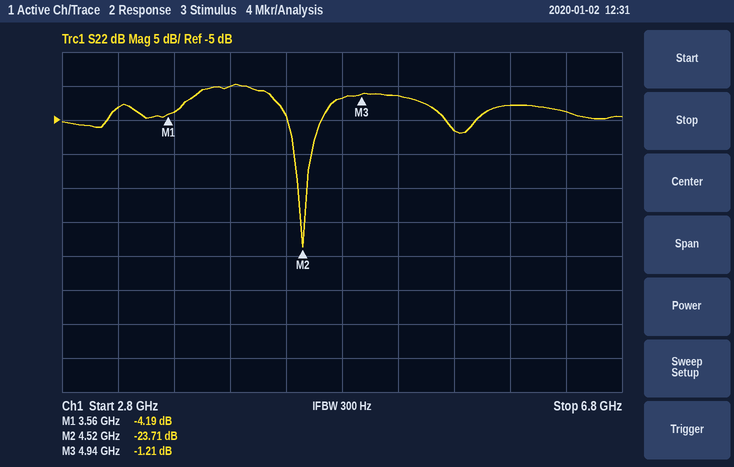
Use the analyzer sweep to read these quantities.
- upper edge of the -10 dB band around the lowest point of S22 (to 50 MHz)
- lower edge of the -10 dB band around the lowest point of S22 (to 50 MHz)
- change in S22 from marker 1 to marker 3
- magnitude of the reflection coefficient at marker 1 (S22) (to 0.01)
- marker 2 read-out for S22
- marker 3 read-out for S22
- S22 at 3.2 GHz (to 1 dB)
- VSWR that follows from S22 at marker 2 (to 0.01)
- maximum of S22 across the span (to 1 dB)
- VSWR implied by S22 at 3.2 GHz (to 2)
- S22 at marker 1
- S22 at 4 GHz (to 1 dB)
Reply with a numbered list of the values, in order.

1. 4.60 GHz
2. 4.45 GHz
3. 2.98 dB
4. 0.62
5. -23.71 dB
6. -1.21 dB
7. -3 dB
8. 1.14
9. 0 dB
10. 6
11. -4.19 dB
12. 0 dB
